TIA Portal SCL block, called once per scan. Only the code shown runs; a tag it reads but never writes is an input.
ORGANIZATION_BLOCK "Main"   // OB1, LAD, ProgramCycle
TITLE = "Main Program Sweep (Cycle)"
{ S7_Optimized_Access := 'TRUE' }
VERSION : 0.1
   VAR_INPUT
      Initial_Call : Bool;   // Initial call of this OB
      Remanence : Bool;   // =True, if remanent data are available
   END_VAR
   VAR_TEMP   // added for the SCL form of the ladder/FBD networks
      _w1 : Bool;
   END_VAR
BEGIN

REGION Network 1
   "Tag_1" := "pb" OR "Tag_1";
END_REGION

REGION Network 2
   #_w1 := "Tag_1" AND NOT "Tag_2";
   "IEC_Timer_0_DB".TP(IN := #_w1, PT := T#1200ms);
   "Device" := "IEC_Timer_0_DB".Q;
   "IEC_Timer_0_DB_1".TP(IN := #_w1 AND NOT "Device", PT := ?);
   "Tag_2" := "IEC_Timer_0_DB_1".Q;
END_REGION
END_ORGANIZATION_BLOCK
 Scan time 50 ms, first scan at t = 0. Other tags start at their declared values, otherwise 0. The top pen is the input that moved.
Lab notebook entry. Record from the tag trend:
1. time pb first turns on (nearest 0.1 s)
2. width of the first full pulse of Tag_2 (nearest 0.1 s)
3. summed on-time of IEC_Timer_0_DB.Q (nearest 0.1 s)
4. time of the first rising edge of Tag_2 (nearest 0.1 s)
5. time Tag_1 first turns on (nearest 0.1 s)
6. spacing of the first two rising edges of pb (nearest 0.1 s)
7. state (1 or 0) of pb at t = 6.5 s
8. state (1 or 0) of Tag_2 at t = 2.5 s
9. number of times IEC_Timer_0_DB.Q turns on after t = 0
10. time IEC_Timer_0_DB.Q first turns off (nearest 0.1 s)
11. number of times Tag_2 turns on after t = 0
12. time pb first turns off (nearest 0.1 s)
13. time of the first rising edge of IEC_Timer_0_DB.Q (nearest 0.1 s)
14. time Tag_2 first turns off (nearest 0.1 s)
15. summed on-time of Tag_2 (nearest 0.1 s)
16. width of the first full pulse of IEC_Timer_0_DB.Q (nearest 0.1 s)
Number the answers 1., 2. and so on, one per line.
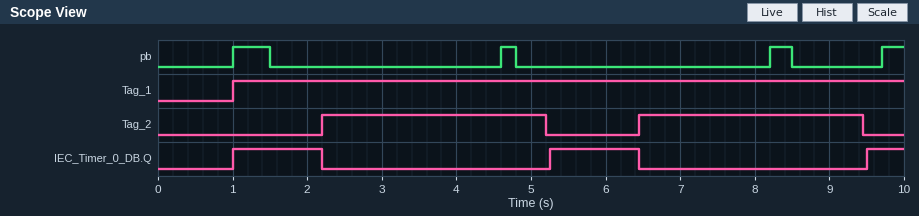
1. 1.0 s
2. 3.0 s
3. 2.9 s
4. 2.2 s
5. 1.0 s
6. 3.6 s
7. 0
8. 1
9. 3
10. 2.2 s
11. 2
12. 1.5 s
13. 1.0 s
14. 5.2 s
15. 6.0 s
16. 1.2 s
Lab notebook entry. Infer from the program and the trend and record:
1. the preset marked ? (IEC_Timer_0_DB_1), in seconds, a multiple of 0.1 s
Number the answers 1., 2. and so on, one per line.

1. 3.0 s
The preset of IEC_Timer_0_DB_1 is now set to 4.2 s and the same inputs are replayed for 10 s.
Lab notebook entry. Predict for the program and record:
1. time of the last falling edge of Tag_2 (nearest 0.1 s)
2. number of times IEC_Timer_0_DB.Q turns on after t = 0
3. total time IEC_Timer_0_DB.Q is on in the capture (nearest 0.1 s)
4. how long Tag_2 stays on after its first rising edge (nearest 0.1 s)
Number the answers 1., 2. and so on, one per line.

1. 6.4 s
2. 2
3. 2.4 s
4. 4.2 s
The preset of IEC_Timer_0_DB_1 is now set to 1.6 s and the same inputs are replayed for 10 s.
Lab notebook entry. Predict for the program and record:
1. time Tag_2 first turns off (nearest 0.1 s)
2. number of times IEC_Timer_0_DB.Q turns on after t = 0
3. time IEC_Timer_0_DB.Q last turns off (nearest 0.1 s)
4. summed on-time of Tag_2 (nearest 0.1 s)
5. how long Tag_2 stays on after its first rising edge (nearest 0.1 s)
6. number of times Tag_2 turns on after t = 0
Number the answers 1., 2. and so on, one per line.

1. 3.8 s
2. 4
3. 7.9 s
4. 4.8 s
5. 1.6 s
6. 3
